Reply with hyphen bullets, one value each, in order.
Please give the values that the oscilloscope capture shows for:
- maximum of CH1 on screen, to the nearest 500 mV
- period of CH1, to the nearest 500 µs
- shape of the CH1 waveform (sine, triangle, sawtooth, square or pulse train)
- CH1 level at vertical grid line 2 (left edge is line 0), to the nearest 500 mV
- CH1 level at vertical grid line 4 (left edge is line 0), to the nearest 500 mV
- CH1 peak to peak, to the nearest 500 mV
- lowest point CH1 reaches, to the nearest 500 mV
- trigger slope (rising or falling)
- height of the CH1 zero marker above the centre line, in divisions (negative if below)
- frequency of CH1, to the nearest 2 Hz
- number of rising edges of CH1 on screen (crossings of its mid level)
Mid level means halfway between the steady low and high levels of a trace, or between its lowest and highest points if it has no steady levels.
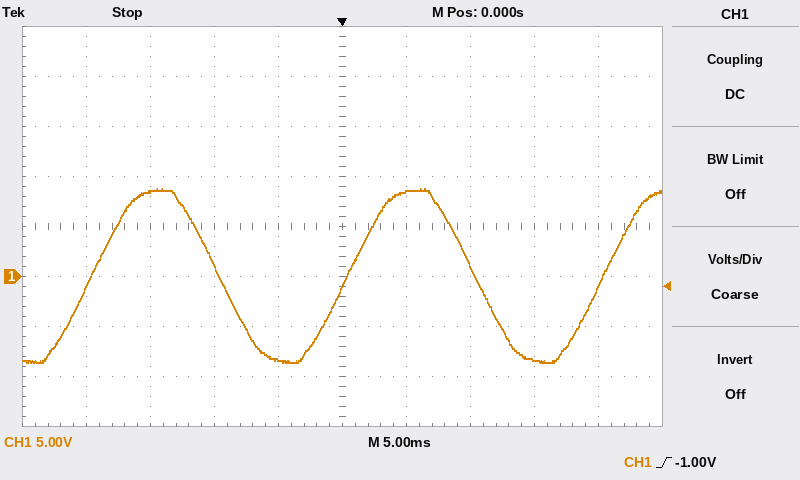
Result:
- 9.0 V
- 20.0 ms
- sine
- 8.5 V
- -8.5 V
- 17.5 V
- -8.5 V
- rising
- -1.0 div
- 50 Hz
- 3
